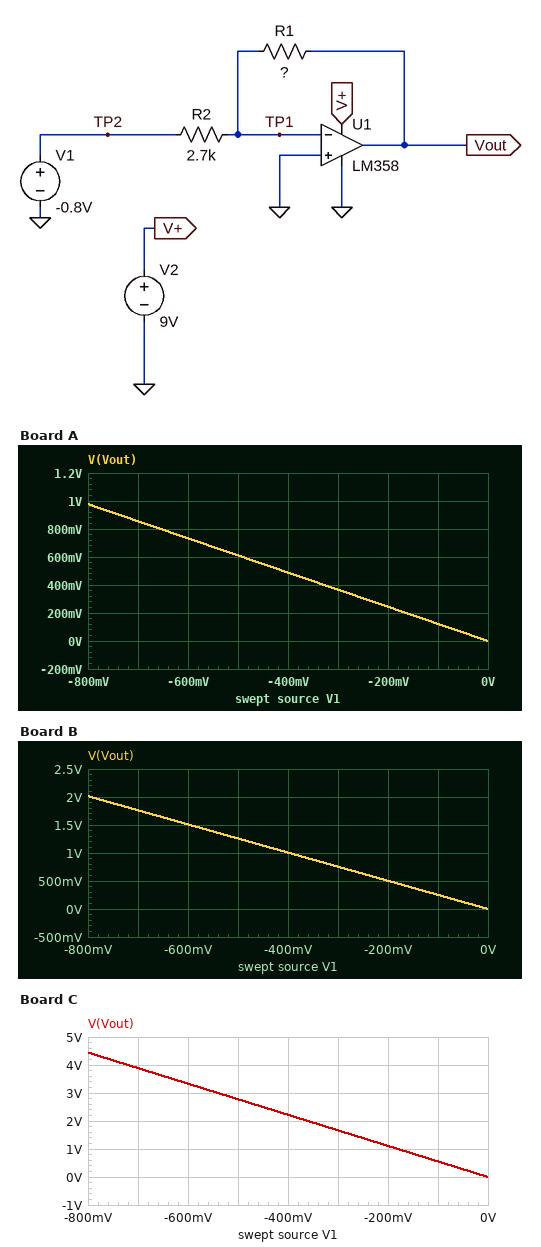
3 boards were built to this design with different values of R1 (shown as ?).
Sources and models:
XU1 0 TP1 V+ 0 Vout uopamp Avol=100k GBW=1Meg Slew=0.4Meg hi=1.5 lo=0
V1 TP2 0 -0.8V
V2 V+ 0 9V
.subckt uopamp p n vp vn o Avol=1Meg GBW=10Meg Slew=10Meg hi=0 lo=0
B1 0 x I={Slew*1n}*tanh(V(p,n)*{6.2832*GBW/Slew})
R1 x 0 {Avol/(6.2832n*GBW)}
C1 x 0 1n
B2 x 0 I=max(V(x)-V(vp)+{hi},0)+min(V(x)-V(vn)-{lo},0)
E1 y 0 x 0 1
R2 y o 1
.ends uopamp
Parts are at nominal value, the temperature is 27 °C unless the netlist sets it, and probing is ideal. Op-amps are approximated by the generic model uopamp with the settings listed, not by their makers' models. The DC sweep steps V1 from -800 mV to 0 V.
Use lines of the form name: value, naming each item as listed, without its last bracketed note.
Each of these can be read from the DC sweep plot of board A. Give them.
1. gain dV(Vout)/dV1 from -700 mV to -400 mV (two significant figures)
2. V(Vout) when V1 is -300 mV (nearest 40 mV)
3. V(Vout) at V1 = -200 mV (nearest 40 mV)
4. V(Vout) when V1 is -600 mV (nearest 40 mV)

gain dV(Vout)/dV1 from -700 mV to -400 mV: -1.2 V/V
V(Vout) when V1 is -300 mV: 360 mV
V(Vout) at V1 = -200 mV: 240 mV
V(Vout) when V1 is -600 mV: 720 mV
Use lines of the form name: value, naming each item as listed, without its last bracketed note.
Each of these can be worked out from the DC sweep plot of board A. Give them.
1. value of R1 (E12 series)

value of R1: 3.3 kΩ
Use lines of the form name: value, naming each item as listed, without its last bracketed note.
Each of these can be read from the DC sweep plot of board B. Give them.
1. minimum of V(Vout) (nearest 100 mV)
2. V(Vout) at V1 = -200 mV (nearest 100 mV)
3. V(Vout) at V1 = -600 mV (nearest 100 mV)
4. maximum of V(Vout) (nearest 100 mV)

minimum of V(Vout): 0 V
V(Vout) at V1 = -200 mV: 500 mV
V(Vout) at V1 = -600 mV: 1.5 V
maximum of V(Vout): 2.0 V
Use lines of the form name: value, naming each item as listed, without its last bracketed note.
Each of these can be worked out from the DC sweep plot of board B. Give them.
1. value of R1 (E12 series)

value of R1: 6.8 kΩ
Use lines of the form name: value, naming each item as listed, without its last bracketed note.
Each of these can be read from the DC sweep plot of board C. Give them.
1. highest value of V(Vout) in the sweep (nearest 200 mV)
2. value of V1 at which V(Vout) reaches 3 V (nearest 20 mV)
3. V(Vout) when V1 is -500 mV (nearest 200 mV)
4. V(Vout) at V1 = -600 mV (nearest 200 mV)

highest value of V(Vout) in the sweep: 4.4 V
value of V1 at which V(Vout) reaches 3 V: -540 mV
V(Vout) when V1 is -500 mV: 2.8 V
V(Vout) at V1 = -600 mV: 3.4 V
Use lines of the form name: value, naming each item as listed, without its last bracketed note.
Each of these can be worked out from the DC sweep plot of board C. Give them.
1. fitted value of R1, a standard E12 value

fitted value of R1, a standard E12 value: 15 kΩ
